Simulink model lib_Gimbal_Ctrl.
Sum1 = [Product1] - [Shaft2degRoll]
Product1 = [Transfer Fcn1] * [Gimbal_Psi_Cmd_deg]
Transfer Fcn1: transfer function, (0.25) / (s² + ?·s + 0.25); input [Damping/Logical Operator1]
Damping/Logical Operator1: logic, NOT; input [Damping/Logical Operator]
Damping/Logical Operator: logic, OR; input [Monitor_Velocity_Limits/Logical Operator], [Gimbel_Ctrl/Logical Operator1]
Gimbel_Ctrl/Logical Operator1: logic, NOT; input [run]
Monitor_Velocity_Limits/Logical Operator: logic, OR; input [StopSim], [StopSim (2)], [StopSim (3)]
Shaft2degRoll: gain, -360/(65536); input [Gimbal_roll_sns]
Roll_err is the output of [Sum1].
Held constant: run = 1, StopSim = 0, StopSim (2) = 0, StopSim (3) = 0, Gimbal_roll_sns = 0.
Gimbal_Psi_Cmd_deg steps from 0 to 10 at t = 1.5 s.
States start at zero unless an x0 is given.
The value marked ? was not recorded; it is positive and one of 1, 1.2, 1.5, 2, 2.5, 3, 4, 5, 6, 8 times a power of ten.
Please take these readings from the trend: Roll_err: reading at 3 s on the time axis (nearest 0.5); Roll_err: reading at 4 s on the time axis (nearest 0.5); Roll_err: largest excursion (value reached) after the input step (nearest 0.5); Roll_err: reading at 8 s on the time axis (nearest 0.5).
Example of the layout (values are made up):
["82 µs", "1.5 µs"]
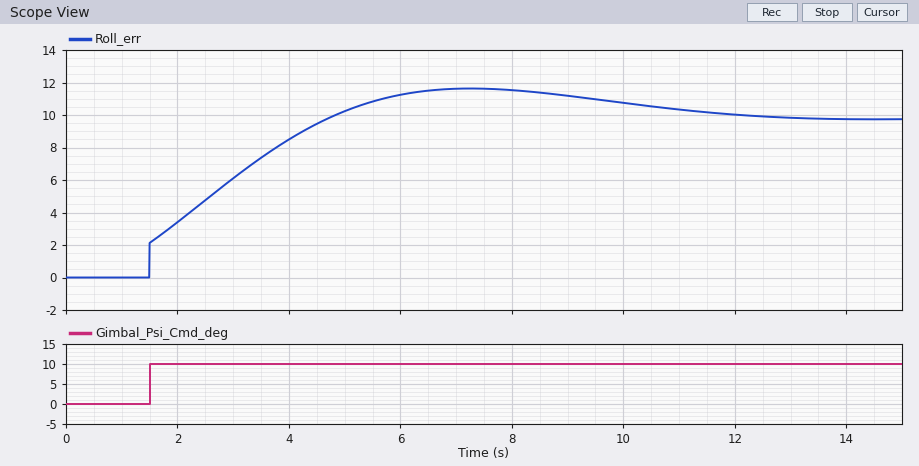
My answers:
["6.0", "8.5", "11.5", "11.5"]
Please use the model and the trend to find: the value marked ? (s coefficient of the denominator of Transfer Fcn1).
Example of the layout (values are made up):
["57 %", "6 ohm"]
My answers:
["0.5"]
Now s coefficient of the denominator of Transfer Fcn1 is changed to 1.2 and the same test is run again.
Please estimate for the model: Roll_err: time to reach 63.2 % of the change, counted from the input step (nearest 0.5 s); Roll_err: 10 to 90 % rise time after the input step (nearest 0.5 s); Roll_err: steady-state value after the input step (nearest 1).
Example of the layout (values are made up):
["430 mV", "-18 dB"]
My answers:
["3.5 s", "8.5 s", "10"]
